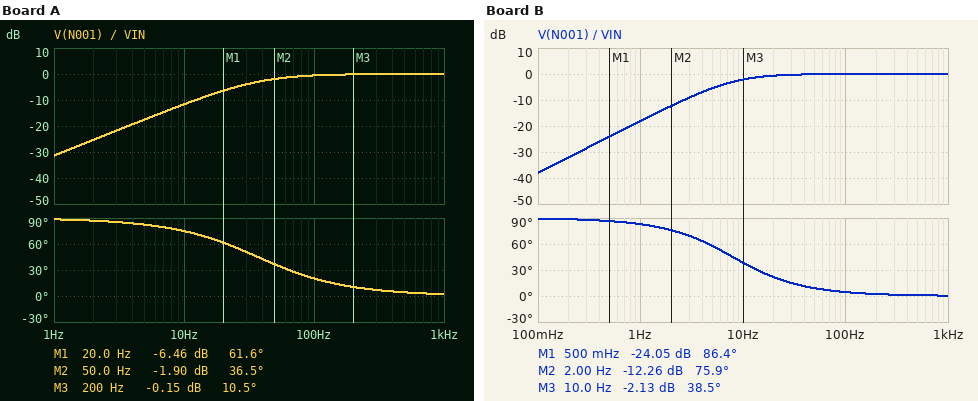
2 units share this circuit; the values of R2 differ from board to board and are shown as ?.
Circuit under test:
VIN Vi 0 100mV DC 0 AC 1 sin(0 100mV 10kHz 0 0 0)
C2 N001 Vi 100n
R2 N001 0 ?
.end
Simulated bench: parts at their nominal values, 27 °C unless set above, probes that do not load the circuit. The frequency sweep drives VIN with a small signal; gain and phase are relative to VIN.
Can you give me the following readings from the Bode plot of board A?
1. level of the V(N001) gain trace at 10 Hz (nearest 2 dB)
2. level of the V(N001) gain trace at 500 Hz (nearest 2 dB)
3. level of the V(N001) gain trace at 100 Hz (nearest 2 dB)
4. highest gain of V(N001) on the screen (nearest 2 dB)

-12 dB
0 dB
0 dB
0 dB
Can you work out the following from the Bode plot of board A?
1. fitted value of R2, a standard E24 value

43 kΩ
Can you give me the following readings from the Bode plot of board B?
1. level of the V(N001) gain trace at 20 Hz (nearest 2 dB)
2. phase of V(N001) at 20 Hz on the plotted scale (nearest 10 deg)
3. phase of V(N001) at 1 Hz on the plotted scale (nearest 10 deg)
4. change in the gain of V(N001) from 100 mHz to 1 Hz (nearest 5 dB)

0 dB
20 deg
80 deg
20 dB
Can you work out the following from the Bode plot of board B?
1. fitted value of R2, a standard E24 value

200 kΩ
